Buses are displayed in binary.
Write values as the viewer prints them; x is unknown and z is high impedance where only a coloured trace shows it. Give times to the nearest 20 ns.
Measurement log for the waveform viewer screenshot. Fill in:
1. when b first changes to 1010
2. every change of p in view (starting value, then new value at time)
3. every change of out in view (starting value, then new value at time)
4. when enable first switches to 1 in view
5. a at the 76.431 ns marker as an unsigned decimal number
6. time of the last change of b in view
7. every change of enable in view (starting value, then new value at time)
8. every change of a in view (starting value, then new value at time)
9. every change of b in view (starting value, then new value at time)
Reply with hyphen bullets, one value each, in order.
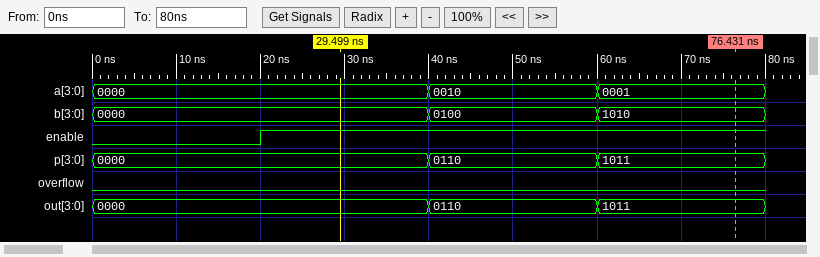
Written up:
- 60 ns
- 0000, 0110 at 40 ns, 1011 at 60 ns
- 0000, 0110 at 40 ns, 1011 at 60 ns
- 20 ns
- 1
- 60 ns
- 0, 1 at 20 ns
- 0000, 0010 at 40 ns, 0001 at 60 ns
- 0000, 0100 at 40 ns, 1010 at 60 ns
